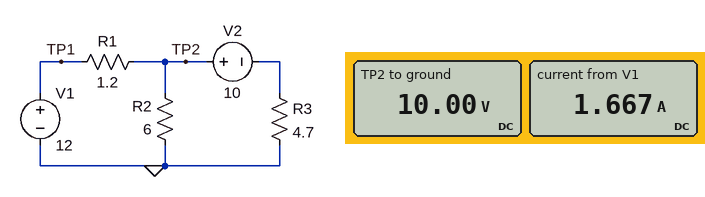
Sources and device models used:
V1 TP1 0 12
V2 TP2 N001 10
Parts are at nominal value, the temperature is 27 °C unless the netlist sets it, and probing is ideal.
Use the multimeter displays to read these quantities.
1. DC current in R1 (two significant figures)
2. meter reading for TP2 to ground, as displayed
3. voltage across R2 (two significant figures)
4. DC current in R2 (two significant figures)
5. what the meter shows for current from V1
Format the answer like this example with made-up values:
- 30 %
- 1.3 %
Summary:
- 1.7 A
- 10.00 V
- 10 V
- 1.7 A
- 1.667 A
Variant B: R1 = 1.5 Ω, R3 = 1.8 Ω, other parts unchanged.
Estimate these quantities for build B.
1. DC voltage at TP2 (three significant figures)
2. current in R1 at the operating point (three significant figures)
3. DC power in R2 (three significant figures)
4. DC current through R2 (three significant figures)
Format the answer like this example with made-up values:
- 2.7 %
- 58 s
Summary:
- 9.76 V
- 1.49 A
- 15.9 W
- 1.63 A
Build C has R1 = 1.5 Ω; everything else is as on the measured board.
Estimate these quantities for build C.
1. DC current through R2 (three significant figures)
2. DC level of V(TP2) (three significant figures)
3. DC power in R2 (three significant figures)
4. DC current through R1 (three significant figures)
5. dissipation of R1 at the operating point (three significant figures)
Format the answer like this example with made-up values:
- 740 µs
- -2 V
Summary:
- 1.61 A
- 9.68 V
- 15.6 W
- 1.55 A
- 3.58 W
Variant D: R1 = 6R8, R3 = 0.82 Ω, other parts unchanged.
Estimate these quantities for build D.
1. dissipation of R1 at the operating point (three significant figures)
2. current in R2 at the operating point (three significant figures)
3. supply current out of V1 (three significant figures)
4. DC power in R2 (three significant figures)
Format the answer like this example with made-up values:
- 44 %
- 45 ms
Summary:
- 1.23 W
- 1.52 A
- 426 mA
- 13.8 W
